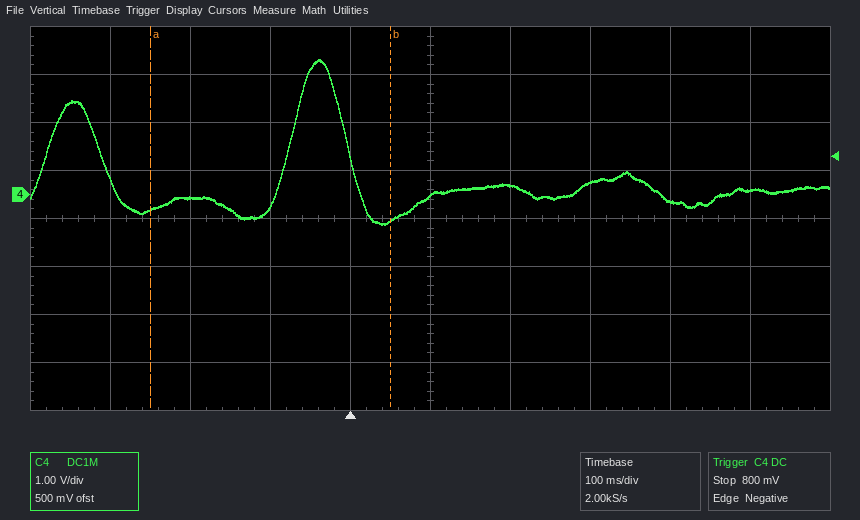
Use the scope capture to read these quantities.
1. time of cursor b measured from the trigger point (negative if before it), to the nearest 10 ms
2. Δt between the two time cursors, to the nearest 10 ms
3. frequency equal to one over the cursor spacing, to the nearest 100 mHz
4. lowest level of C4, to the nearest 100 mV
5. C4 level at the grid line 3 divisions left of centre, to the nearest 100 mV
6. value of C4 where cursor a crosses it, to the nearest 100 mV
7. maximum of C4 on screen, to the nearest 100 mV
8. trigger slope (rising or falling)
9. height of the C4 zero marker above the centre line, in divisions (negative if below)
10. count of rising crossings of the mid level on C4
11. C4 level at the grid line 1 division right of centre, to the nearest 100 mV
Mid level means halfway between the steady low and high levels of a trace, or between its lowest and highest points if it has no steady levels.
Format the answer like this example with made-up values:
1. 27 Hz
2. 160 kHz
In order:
1. +50 ms
2. 300 ms
3. 3.3 Hz
4. -600 mV
5. -100 mV
6. -300 mV
7. 2.8 V
8. falling
9. +0.5 div
10. 2
11. 200 mV
